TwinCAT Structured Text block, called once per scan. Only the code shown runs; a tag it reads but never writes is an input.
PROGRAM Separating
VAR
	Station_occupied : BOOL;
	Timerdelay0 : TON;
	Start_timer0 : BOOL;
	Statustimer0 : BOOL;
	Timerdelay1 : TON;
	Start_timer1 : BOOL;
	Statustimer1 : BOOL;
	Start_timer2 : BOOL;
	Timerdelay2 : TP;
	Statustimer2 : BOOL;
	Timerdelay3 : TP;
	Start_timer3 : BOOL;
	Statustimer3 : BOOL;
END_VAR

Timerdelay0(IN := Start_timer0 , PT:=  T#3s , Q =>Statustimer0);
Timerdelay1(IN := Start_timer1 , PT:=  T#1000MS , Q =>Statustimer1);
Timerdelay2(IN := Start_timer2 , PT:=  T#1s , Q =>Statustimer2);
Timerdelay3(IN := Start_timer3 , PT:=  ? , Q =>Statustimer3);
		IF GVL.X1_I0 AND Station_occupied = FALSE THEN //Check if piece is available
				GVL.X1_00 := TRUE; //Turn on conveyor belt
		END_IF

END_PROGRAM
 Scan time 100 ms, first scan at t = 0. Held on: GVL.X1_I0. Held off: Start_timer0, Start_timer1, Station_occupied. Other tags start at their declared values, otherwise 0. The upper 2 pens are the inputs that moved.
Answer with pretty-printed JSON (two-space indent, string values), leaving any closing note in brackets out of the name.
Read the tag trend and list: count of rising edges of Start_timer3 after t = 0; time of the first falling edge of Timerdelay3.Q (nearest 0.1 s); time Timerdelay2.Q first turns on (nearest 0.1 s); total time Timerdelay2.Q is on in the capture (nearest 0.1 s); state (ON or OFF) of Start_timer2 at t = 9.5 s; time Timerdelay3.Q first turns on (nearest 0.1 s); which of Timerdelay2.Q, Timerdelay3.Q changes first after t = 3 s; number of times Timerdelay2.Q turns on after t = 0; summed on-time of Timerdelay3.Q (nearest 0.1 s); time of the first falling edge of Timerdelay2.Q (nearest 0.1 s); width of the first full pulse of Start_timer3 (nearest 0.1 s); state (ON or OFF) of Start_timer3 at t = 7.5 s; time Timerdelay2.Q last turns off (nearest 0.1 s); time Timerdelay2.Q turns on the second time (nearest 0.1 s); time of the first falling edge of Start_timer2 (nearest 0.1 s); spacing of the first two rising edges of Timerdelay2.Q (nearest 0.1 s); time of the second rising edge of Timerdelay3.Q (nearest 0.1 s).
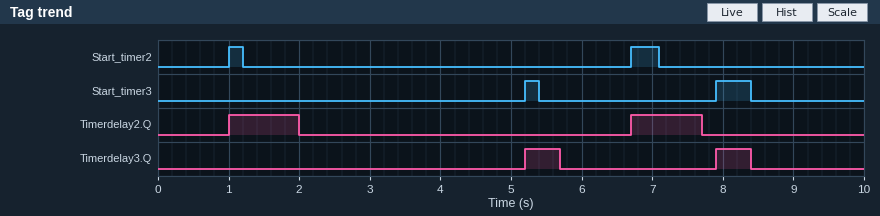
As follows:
{
  "count of rising edges of Start_timer3 after t = 0": "2",
  "time of the first falling edge of Timerdelay3.Q": "5.7 s",
  "time Timerdelay2.Q first turns on": "1.0 s",
  "total time Timerdelay2.Q is on in the capture": "2.0 s",
  "state (ON or OFF) of Start_timer2 at t = 9.5 s": "OFF",
  "time Timerdelay3.Q first turns on": "5.2 s",
  "which of Timerdelay2.Q, Timerdelay3.Q changes first after t = 3 s": "Timerdelay3.Q",
  "number of times Timerdelay2.Q turns on after t = 0": "2",
  "summed on-time of Timerdelay3.Q": "1.0 s",
  "time of the first falling edge of Timerdelay2.Q": "2.0 s",
  "width of the first full pulse of Start_timer3": "0.2 s",
  "state (ON or OFF) of Start_timer3 at t = 7.5 s": "OFF",
  "time Timerdelay2.Q last turns off": "7.7 s",
  "time Timerdelay2.Q turns on the second time": "6.7 s",
  "time of the first falling edge of Start_timer2": "1.2 s",
  "spacing of the first two rising edges of Timerdelay2.Q": "5.7 s",
  "time of the second rising edge of Timerdelay3.Q": "7.9 s"
}
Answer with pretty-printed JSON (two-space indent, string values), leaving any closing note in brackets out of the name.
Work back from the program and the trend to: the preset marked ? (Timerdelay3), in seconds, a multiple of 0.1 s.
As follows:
{
  "the preset marked ? (Timerdelay3), in seconds, a multiple of 0.1 s": "0.5 s"
}
